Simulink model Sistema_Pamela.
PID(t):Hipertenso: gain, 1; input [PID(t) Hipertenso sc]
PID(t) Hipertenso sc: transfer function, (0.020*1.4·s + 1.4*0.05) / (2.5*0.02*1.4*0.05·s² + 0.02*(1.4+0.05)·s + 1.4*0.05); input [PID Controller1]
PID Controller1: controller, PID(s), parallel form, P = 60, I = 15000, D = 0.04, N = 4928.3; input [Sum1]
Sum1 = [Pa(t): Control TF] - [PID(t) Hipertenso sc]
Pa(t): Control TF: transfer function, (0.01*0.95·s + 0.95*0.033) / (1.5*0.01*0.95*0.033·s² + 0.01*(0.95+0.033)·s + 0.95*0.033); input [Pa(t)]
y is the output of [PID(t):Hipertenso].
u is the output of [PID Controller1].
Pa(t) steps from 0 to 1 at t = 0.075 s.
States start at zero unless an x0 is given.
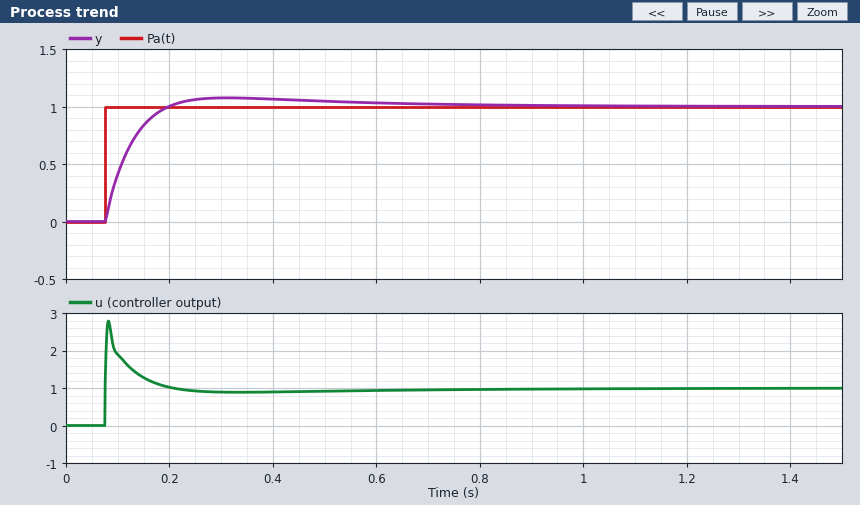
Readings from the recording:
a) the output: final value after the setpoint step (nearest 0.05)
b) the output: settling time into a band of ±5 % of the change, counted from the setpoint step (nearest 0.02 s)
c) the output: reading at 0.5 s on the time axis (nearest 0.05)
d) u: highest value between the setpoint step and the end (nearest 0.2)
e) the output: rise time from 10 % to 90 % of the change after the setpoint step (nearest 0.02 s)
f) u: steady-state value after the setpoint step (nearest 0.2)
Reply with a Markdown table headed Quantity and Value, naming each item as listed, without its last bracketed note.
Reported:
| Quantity | Value |
|---|---|
| the output: final value after the setpoint step | 1.00 |
| the output: settling time into a band of ±5 % of the change, counted from the setpoint step | 0.40 s |
| the output: reading at 0.5 s on the time axis | 1.05 |
| u: highest value between the setpoint step and the end | 2.8 |
| the output: rise time from 10 % to 90 % of the change after the setpoint step | 0.08 s |
| u: steady-state value after the setpoint step | 1.0 |
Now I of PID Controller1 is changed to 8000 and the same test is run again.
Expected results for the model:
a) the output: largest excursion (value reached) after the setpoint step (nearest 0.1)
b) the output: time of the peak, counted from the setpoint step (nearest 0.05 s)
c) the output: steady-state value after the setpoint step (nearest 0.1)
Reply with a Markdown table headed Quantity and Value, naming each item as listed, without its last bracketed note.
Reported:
| Quantity | Value |
|---|---|
| the output: largest excursion (value reached) after the setpoint step | 1.1 |
| the output: time of the peak, counted from the setpoint step | 0.25 s |
| the output: steady-state value after the setpoint step | 1.0 |
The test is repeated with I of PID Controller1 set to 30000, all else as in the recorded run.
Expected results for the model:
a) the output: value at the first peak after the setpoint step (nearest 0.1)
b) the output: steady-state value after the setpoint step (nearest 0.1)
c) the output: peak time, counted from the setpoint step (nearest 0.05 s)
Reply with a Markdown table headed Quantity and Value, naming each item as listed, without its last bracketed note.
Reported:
| Quantity | Value |
|---|---|
| the output: value at the first peak after the setpoint step | 1.1 |
| the output: steady-state value after the setpoint step | 1.0 |
| the output: peak time, counted from the setpoint step | 0.25 s |
